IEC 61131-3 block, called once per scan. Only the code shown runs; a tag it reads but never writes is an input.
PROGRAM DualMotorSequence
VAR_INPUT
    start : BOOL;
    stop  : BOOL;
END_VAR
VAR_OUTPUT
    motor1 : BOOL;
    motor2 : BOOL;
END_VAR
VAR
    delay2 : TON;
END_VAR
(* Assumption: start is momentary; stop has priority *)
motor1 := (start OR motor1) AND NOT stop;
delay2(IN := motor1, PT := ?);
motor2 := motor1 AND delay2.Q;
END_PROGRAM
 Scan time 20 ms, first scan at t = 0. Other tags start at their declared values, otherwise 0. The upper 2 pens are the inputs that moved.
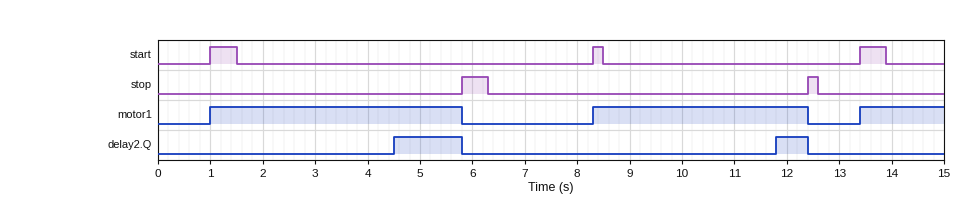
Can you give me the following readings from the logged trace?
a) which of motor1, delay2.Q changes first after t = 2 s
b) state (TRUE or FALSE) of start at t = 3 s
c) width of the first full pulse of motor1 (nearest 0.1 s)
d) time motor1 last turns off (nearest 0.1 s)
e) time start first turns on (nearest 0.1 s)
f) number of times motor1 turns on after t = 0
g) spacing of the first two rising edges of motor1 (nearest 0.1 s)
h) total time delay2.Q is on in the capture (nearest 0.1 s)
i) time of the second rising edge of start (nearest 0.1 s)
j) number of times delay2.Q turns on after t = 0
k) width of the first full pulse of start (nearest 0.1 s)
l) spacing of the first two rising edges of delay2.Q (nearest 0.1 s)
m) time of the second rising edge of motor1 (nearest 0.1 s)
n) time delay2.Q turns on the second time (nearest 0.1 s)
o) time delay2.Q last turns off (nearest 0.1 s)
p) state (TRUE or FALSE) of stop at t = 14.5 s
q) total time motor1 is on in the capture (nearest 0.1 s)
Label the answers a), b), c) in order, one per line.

a) delay2.Q
b) FALSE
c) 4.8 s
d) 12.4 s
e) 1.0 s
f) 3
g) 7.3 s
h) 1.9 s
i) 8.3 s
j) 2
k) 0.5 s
l) 7.3 s
m) 8.3 s
n) 11.8 s
o) 12.4 s
p) FALSE
q) 10.5 s
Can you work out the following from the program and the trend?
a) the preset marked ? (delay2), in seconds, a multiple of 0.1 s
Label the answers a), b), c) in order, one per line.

a) 3.5 s
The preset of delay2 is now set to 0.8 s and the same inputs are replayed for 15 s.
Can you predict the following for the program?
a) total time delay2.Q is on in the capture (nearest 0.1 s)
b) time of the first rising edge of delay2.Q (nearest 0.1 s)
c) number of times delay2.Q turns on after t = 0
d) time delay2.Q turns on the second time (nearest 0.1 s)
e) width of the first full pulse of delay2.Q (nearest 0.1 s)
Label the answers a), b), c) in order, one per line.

a) 8.1 s
b) 1.8 s
c) 3
d) 9.1 s
e) 4.0 s
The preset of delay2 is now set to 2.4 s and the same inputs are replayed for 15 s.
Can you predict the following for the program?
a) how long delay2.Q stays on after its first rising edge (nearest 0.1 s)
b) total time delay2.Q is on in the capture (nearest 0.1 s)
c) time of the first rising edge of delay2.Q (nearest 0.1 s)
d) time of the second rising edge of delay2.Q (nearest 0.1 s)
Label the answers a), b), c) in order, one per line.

a) 2.4 s
b) 4.1 s
c) 3.4 s
d) 10.7 s
